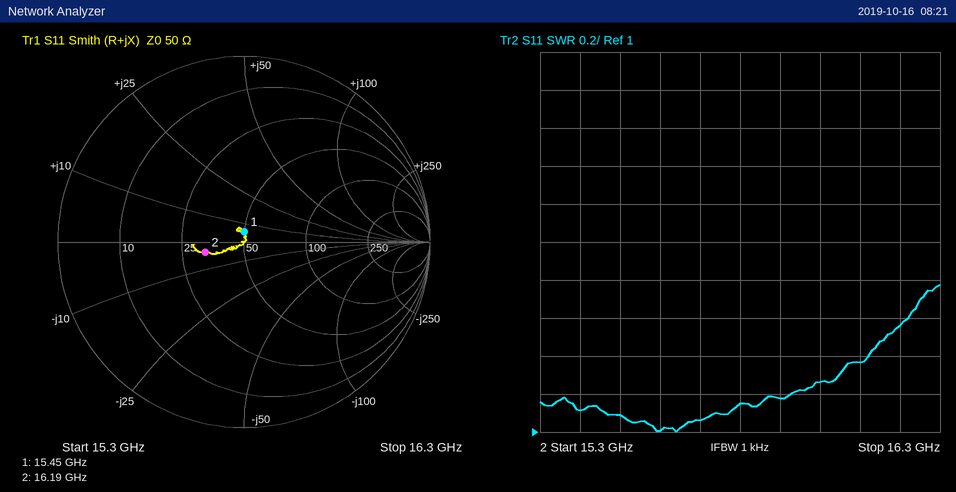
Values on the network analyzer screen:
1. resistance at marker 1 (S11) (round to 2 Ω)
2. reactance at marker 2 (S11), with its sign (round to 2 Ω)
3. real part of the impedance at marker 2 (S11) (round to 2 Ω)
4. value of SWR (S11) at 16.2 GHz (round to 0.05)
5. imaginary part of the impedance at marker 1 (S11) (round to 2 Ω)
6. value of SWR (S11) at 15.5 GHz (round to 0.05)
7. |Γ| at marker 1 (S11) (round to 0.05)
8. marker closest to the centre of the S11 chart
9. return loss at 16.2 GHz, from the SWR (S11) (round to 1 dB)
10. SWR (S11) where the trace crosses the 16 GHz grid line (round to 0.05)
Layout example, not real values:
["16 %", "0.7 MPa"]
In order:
["50 Ω", "-4 Ω", "32 Ω", "1.55", "+6 Ω", "1.10", "0.05", "marker 1", "13 dB", "1.25"]
